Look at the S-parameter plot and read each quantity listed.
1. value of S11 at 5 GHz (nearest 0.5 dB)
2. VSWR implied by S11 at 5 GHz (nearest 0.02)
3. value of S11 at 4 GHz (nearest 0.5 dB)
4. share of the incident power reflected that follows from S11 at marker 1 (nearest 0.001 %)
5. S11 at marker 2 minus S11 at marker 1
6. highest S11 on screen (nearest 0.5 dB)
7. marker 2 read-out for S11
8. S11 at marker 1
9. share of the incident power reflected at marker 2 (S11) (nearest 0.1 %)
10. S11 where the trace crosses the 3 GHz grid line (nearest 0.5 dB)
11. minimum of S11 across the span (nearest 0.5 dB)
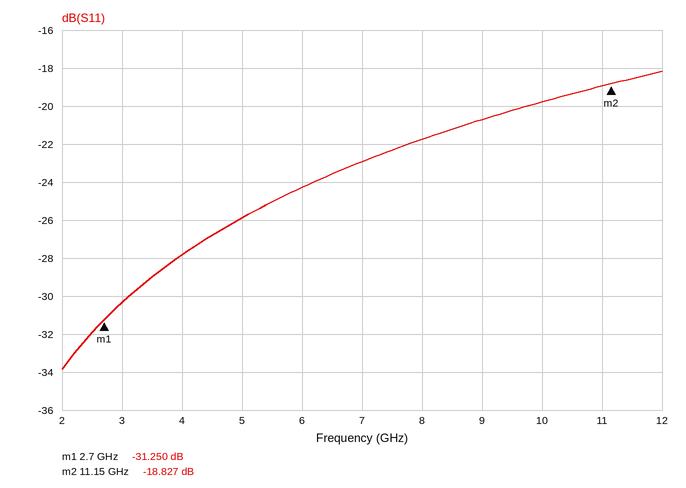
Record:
-26.0 dB
1.10
-28.0 dB
0.075 %
12.423 dB
-18.0 dB
-18.827 dB
-31.250 dB
1.3 %
-30.5 dB
-34.0 dB
